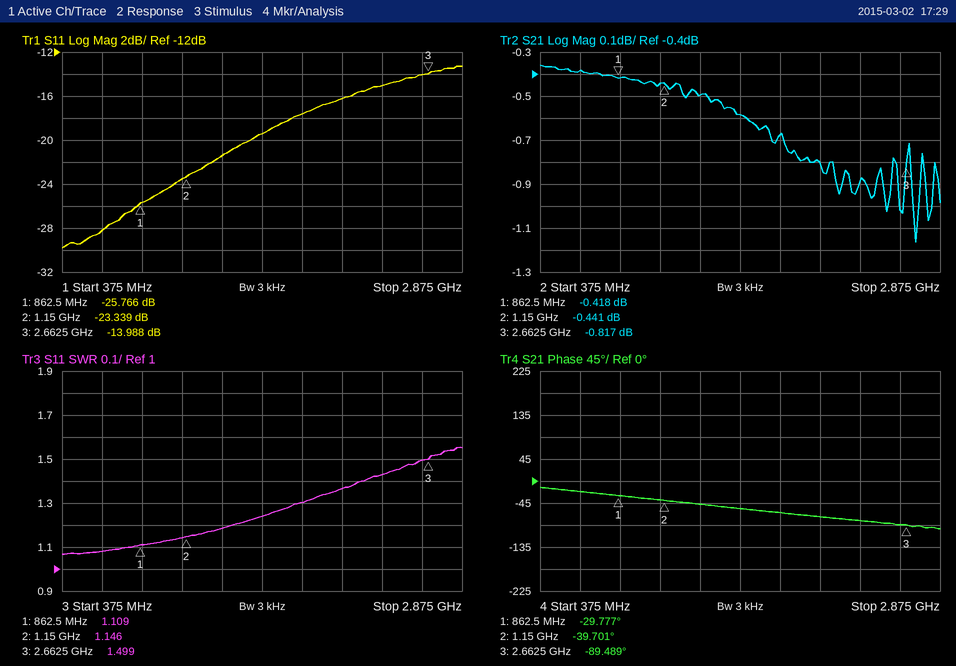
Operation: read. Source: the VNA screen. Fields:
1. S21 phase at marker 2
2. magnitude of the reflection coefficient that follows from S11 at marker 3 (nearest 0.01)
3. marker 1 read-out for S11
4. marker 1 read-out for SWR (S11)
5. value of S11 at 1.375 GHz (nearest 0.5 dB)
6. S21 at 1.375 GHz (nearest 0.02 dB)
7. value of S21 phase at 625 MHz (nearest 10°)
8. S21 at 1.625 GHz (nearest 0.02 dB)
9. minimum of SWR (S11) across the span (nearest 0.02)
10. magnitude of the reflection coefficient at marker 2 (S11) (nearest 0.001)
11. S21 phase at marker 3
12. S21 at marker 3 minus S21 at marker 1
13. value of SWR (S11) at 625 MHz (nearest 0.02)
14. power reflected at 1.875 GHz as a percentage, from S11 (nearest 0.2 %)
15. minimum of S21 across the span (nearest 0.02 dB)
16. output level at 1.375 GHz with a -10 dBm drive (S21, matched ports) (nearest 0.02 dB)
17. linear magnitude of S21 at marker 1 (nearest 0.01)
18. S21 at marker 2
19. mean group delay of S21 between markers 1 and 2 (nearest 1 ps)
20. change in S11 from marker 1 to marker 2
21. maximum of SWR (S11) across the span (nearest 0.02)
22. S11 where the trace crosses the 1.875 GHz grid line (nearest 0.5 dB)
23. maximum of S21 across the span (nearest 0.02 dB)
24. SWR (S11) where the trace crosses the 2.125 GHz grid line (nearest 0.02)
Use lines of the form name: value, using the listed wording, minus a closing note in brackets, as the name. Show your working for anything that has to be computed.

S21 phase at marker 2: -39.701°
magnitude of the reflection coefficient that follows from S11 at marker 3: 10^(-13.988/20) ≈ 0.20
marker 1 read-out for S11: -25.766 dB
marker 1 read-out for SWR: 1.109
value of S11 at 1.375 GHz: -21.5 dB
S21 at 1.375 GHz: -0.50 dB
value of S21 phase at 625 MHz: -20°
S21 at 1.625 GHz: -0.58 dB
minimum of SWR (S11) across the span: 1.06
magnitude of the reflection coefficient at marker 2 (S11): 10^(-23.339/20) ≈ 0.068
S21 phase at marker 3: -89.489°
S21 at marker 3 minus S21 at marker 1: -0.817 − (-0.418) = -0.399 dB
value of SWR (S11) at 625 MHz: 1.08
power reflected at 1.875 GHz as a percentage, from S11: 10^(-17.5/10) ≈ 1.8 %
minimum of S21 across the span: -1.16 dB
output level at 1.375 GHz with a -10 dBm drive (S21, matched ports): -10 dBm + (-0.50 dB) = -10.50 dBm
linear magnitude of S21 at marker 1: 10^(-0.418/20) ≈ 0.95
S21 at marker 2: -0.441 dB
mean group delay of S21 between markers 1 and 2: −(-39.701° − (-29.777°))/(360° × 287.5 MHz) ≈ 96 ps
change in S11 from marker 1 to marker 2: -23.339 − (-25.766) = 2.427 dB
maximum of SWR (S11) across the span: 1.56
S11 where the trace crosses the 1.875 GHz grid line: -17.5 dB
maximum of S21 across the span: -0.36 dB
SWR (S11) where the trace crosses the 2.125 GHz grid line: 1.36
